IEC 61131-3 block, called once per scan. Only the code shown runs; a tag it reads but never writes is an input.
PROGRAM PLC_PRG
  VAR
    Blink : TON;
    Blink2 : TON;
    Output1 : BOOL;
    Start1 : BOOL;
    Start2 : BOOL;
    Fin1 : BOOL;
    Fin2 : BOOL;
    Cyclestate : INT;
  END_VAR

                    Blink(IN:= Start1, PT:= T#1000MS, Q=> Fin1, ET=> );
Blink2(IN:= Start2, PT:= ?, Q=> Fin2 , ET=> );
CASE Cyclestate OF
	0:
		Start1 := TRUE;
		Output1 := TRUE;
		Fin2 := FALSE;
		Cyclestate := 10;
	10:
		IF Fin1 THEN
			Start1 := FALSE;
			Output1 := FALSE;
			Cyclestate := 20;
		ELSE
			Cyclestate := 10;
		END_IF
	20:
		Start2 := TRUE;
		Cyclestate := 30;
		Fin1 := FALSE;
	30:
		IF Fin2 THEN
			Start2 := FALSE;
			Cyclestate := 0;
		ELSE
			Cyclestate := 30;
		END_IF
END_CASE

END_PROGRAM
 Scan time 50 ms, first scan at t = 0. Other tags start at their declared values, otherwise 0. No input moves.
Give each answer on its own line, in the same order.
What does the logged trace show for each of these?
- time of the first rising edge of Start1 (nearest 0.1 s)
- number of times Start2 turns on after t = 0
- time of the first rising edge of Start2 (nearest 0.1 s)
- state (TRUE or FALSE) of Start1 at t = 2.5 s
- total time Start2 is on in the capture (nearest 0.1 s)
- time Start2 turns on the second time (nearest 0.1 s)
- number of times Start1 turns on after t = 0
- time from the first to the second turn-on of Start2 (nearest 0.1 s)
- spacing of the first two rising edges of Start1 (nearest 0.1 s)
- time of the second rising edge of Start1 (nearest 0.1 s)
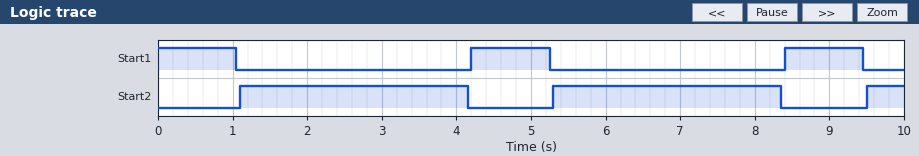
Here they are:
4.2 s
3
1.1 s
FALSE
6.6 s
5.3 s
2
4.2 s
4.2 s
8.4 s
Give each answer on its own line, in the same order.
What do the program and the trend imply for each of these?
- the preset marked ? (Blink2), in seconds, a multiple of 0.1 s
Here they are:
3.0 s
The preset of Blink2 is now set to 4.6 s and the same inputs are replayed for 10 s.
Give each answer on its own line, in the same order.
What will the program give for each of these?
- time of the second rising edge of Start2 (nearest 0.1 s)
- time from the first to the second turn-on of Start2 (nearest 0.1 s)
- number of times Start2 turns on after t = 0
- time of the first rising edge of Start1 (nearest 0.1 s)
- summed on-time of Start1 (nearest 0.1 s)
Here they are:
6.9 s
5.8 s
2
5.8 s
2.1 s
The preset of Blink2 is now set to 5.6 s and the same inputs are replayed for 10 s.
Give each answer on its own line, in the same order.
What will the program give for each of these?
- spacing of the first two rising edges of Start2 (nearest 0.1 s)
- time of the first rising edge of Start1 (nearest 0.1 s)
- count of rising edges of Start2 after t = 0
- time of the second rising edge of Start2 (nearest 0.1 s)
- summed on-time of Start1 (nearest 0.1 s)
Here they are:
6.8 s
6.8 s
2
7.9 s
2.1 s
